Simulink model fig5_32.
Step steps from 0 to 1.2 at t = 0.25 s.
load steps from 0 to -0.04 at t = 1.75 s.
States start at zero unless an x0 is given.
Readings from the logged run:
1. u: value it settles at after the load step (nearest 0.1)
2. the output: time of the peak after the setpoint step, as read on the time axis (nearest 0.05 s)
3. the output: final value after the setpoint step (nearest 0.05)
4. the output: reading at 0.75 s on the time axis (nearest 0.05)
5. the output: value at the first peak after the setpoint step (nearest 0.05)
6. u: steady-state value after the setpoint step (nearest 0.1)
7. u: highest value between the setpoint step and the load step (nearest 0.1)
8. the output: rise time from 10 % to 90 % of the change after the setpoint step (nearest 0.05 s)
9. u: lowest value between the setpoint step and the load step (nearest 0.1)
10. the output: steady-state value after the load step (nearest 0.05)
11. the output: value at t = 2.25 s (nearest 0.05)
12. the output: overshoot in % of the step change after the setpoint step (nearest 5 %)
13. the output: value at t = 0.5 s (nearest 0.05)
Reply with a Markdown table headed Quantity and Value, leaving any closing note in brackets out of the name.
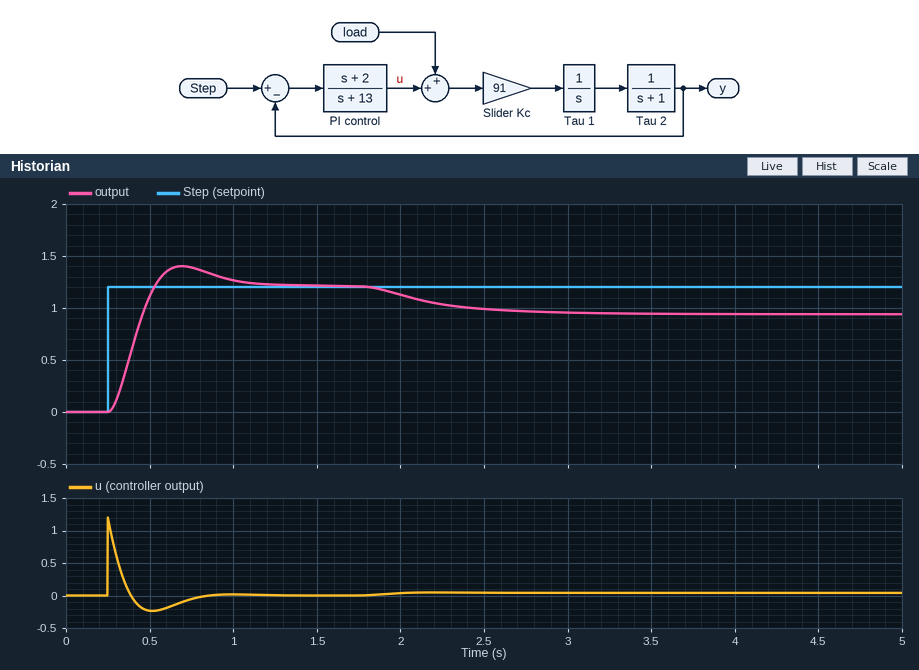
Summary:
| Quantity | Value |
|---|---|
| u: value it settles at after the load step | 0.0 |
| the output: time of the peak after the setpoint step, as read on the time axis | 0.70 s |
| the output: final value after the setpoint step | 1.20 |
| the output: reading at 0.75 s on the time axis | 1.40 |
| the output: value at the first peak after the setpoint step | 1.40 |
| u: steady-state value after the setpoint step | 0.0 |
| u: highest value between the setpoint step and the load step | 1.2 |
| the output: rise time from 10 % to 90 % of the change after the setpoint step | 0.20 s |
| u: lowest value between the setpoint step and the load step | -0.2 |
| the output: steady-state value after the load step | 0.95 |
| the output: value at t = 2.25 s | 1.05 |
| the output: overshoot in % of the step change after the setpoint step | 15 % |
| the output: value at t = 0.5 s | 1.10 |
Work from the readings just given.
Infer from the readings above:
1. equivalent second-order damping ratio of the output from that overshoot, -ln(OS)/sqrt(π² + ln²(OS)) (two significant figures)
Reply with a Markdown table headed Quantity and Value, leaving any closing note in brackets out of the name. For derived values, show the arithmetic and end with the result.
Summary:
| Quantity | Value |
|---|---|
| equivalent second-order damping ratio of the output from that overshoot, -ln(OS)/sqrt(π² + ln²(OS)) | ln(0.15) = -1.897; 1.897 / sqrt(9.870 + 3.599) = 0.52 |
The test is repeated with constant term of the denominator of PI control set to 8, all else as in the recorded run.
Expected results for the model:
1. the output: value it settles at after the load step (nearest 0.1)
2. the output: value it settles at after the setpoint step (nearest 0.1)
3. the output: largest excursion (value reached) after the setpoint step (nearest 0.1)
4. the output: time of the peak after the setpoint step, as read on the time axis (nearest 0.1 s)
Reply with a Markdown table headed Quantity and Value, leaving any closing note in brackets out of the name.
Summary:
| Quantity | Value |
|---|---|
| the output: value it settles at after the load step | 1.0 |
| the output: value it settles at after the setpoint step | 1.2 |
| the output: largest excursion (value reached) after the setpoint step | 1.6 |
| the output: time of the peak after the setpoint step, as read on the time axis | 0.6 s |
